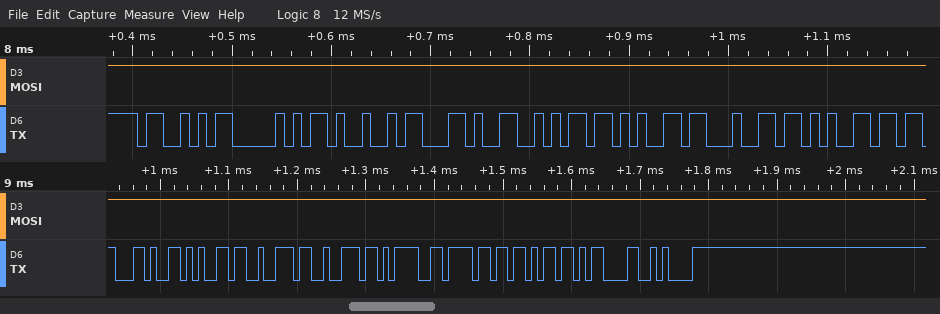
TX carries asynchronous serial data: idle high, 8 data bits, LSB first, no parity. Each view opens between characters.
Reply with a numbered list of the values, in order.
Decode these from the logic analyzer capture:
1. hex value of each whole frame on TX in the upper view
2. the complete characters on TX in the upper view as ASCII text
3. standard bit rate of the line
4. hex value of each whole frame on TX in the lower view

1. 53, 50, 49, 2C, 6A, 65, 64, 65
2. "SPI,jede"
3. 115200 baud
4. 2C, 65, 72, 72, 3D, 6F, 6B, 0D, 0A
